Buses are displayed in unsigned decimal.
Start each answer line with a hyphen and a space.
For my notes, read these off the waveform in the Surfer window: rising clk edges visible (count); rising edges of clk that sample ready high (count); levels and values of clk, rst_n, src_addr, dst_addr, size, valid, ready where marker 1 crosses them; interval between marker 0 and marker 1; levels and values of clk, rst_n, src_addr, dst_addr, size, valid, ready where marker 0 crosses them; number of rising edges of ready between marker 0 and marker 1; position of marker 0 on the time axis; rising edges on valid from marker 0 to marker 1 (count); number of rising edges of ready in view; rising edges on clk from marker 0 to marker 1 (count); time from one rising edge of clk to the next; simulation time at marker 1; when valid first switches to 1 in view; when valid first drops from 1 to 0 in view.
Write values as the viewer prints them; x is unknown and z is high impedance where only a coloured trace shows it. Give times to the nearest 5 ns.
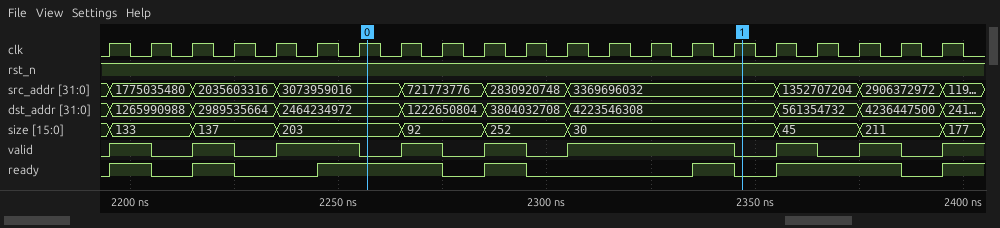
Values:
- 21
- 10
- clk=1, rst_n=1, src_addr=3369696032, dst_addr=4223546308, size=30, valid=0, ready=0
- 90 ns
- clk=1, rst_n=1, src_addr=3073959016, dst_addr=2464234972, size=203, valid=0, ready=1
- 2
- 2255 ns
- 3
- 7
- 9
- 10 ns
- 2345 ns
- 2195 ns
- 2205 ns
